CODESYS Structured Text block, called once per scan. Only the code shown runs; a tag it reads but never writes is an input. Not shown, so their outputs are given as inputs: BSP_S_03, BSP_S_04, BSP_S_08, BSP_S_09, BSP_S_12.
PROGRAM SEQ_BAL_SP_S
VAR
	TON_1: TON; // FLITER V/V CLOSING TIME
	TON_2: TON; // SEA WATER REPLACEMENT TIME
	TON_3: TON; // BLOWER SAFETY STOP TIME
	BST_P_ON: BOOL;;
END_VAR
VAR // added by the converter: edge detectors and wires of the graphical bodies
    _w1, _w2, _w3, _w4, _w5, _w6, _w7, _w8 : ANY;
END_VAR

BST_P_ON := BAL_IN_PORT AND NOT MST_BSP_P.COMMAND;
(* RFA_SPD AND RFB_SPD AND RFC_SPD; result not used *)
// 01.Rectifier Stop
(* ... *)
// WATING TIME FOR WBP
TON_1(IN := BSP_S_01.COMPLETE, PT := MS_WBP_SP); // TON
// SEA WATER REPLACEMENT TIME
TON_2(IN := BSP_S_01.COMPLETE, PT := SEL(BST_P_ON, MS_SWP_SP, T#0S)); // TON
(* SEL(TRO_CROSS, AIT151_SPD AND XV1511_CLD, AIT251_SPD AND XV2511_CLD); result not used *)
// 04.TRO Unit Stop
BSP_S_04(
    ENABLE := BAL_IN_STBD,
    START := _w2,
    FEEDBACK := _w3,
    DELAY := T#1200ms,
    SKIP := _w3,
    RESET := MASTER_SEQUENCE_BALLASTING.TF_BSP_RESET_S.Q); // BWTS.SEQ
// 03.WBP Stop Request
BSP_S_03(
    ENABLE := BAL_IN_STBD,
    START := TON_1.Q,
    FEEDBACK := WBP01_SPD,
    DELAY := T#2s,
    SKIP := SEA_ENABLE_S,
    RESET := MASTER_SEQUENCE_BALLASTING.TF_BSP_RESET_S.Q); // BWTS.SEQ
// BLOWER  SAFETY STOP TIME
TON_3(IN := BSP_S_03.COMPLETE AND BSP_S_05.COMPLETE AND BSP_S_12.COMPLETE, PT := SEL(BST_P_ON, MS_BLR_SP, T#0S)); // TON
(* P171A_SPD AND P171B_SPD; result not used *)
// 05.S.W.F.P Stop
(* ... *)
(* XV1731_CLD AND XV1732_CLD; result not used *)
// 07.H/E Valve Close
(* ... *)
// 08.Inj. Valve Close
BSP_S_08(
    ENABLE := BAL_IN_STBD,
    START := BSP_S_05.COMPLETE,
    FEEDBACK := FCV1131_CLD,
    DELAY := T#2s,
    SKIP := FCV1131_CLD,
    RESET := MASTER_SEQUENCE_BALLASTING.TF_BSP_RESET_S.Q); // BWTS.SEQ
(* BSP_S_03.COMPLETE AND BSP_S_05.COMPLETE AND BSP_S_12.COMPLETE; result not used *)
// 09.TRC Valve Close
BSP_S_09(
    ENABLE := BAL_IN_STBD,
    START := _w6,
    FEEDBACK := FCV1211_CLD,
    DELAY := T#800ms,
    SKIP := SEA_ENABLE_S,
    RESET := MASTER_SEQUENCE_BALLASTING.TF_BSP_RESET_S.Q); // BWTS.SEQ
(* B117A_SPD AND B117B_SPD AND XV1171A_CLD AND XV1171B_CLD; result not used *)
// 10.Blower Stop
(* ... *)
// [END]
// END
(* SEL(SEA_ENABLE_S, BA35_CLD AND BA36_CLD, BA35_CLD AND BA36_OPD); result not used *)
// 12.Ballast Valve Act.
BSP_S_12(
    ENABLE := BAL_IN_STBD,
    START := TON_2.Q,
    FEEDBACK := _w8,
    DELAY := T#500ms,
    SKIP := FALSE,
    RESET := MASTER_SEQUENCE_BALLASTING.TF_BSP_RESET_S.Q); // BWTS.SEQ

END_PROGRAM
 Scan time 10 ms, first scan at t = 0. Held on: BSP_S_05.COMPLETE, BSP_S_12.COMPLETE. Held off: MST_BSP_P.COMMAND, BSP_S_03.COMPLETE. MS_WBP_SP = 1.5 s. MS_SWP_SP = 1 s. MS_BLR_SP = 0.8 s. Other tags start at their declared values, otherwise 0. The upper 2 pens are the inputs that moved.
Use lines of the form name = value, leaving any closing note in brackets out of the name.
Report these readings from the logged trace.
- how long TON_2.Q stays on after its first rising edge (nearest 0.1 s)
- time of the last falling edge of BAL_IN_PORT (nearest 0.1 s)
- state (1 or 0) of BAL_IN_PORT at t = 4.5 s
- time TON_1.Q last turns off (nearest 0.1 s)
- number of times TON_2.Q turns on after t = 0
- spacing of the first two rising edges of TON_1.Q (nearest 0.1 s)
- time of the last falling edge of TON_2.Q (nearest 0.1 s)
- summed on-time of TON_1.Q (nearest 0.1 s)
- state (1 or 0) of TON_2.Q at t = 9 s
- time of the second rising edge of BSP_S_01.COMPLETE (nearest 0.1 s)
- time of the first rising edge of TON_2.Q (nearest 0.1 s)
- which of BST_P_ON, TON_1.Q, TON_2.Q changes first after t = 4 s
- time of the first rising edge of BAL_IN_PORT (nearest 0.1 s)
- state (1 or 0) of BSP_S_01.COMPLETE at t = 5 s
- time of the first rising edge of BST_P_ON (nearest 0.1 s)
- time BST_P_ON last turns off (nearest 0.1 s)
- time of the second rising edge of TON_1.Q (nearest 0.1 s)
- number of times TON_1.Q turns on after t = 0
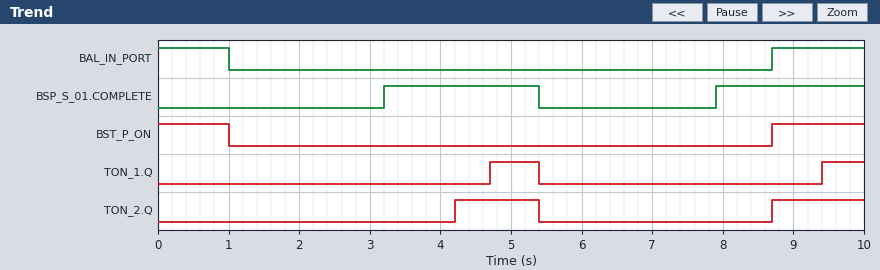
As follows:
how long TON_2.Q stays on after its first rising edge = 1.2 s
time of the last falling edge of BAL_IN_PORT = 1.0 s
state (1 or 0) of BAL_IN_PORT at t = 4.5 s = 0
time TON_1.Q last turns off = 5.4 s
number of times TON_2.Q turns on after t = 0 = 2
spacing of the first two rising edges of TON_1.Q = 4.7 s
time of the last falling edge of TON_2.Q = 5.4 s
summed on-time of TON_1.Q = 1.3 s
state (1 or 0) of TON_2.Q at t = 9 s = 1
time of the second rising edge of BSP_S_01.COMPLETE = 7.9 s
time of the first rising edge of TON_2.Q = 4.2 s
which of BST_P_ON, TON_1.Q, TON_2.Q changes first after t = 4 s = TON_2.Q
time of the first rising edge of BAL_IN_PORT = 8.7 s
state (1 or 0) of BSP_S_01.COMPLETE at t = 5 s = 1
time of the first rising edge of BST_P_ON = 8.7 s
time BST_P_ON last turns off = 1.0 s
time of the second rising edge of TON_1.Q = 9.4 s
number of times TON_1.Q turns on after t = 0 = 2
